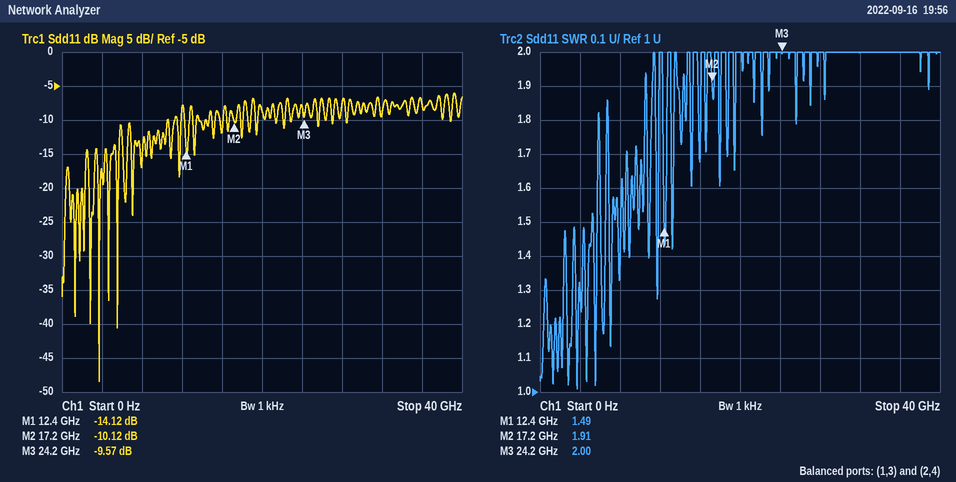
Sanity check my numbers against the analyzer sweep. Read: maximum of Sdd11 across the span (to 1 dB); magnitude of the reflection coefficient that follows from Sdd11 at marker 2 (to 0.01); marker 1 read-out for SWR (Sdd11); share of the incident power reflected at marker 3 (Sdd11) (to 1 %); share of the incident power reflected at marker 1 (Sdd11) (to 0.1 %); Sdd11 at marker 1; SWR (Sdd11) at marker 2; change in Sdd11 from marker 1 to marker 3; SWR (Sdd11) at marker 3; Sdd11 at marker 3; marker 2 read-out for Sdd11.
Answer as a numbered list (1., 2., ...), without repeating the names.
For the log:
1. -6 dB
2. 0.31
3. 1.49
4. 11 %
5. 3.9 %
6. -14.12 dB
7. 1.91
8. 4.55 dB
9. 2.00
10. -9.57 dB
11. -10.12 dB
